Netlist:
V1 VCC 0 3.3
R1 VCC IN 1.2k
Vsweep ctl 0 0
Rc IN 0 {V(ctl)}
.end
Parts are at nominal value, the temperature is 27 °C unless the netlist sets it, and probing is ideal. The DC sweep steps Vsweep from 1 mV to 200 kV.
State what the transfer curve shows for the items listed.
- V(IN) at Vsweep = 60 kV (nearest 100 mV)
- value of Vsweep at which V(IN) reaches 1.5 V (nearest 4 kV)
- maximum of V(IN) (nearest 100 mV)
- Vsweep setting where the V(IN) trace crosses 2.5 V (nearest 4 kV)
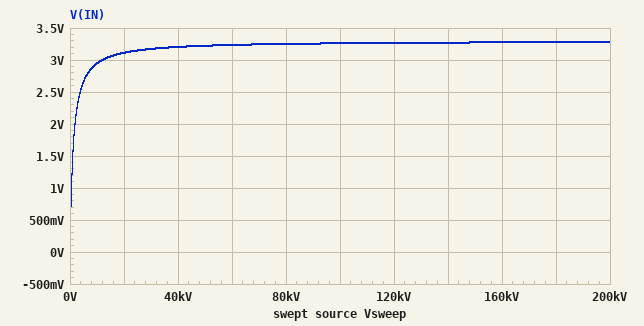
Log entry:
3.2 V
0 V
3.3 V
4 kV
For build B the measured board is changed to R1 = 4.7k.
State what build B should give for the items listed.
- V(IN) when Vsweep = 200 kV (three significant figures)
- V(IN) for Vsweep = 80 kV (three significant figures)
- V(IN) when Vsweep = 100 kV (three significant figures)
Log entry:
3.22 V
3.12 V
3.15 V
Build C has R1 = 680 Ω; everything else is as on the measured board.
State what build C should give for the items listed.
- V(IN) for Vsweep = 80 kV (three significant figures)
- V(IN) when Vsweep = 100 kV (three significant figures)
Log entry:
3.27 V
3.28 V
